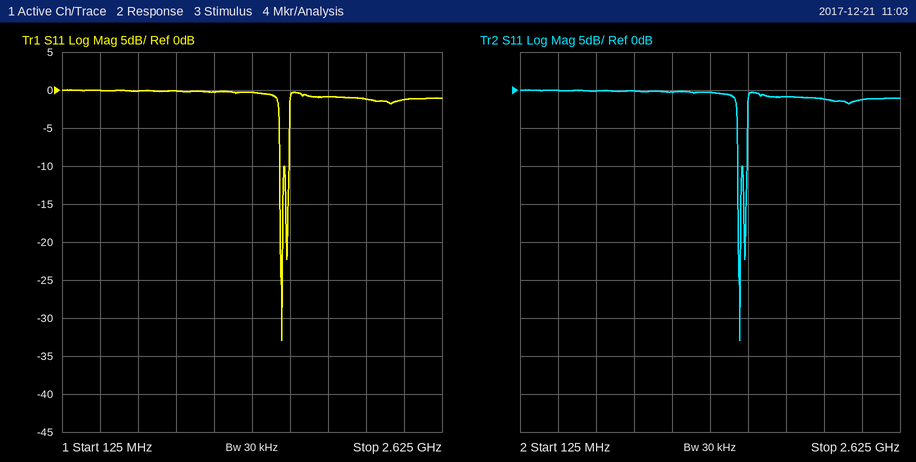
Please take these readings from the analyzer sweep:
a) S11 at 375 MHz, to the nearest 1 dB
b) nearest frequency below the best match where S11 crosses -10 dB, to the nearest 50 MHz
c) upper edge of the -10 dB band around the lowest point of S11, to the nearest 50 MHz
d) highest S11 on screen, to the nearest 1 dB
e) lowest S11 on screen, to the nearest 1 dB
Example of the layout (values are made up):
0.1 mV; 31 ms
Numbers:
0 dB; 1.55 GHz; 1.60 GHz; 0 dB; -33 dB
